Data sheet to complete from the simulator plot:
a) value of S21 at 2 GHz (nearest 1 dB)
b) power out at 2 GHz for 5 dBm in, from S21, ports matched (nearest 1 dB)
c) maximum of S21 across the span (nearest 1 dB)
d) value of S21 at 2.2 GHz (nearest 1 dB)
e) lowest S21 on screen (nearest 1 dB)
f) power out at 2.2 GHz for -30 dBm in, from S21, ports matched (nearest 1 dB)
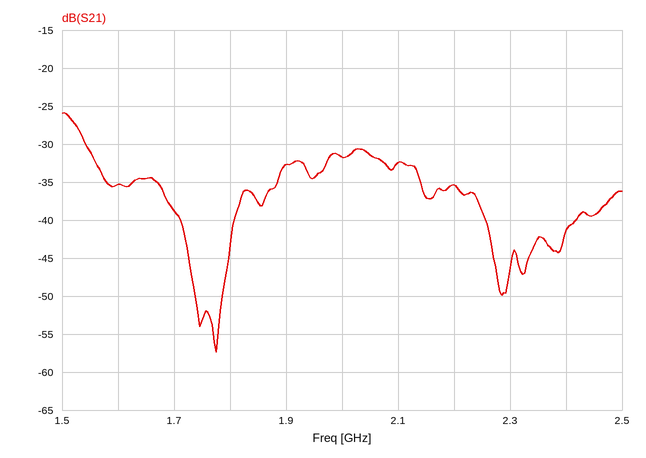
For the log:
-32 dB
-27 dBm
-26 dB
-35 dB
-57 dB
-65 dBm
